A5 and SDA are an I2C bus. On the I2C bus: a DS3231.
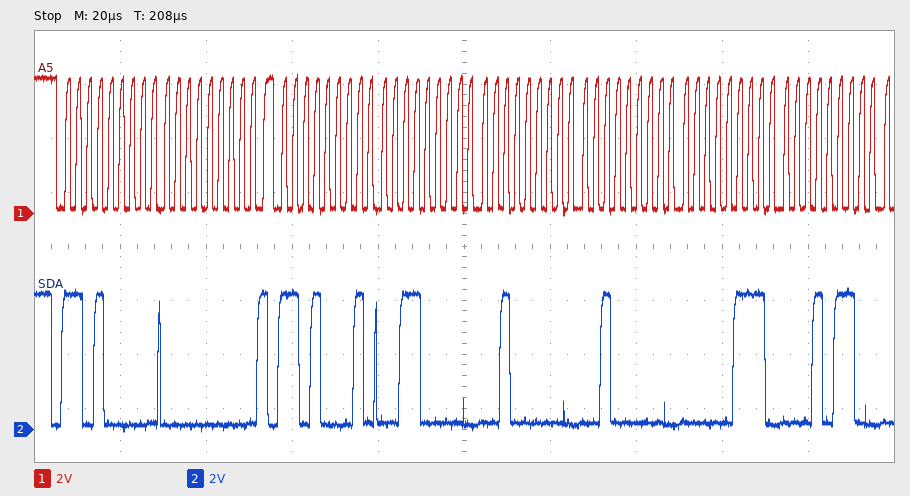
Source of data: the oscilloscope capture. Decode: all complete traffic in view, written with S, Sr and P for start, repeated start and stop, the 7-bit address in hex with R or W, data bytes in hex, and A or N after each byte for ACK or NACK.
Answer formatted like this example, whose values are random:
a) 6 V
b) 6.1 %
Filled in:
a) S 68W A 00 A Sr 68R A 30 A 20 A 20 A 07 A 16 A
